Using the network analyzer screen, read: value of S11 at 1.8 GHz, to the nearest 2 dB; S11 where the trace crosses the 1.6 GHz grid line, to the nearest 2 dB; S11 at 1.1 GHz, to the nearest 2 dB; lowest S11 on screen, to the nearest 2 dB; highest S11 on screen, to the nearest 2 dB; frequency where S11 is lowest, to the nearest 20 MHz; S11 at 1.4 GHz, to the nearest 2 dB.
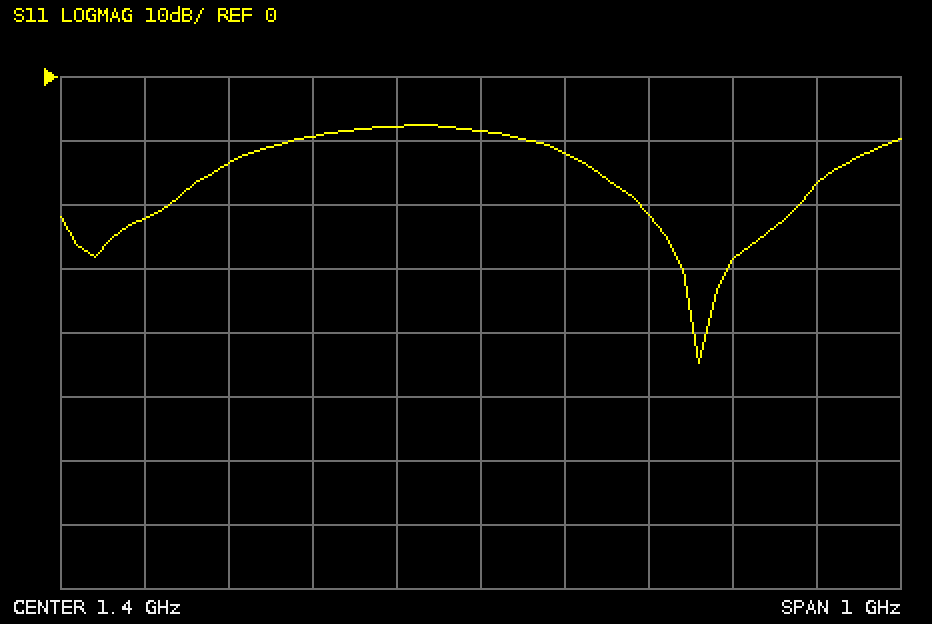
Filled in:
-16 dB
-22 dB
-14 dB
-44 dB
-8 dB
1.66 GHz
-8 dB
